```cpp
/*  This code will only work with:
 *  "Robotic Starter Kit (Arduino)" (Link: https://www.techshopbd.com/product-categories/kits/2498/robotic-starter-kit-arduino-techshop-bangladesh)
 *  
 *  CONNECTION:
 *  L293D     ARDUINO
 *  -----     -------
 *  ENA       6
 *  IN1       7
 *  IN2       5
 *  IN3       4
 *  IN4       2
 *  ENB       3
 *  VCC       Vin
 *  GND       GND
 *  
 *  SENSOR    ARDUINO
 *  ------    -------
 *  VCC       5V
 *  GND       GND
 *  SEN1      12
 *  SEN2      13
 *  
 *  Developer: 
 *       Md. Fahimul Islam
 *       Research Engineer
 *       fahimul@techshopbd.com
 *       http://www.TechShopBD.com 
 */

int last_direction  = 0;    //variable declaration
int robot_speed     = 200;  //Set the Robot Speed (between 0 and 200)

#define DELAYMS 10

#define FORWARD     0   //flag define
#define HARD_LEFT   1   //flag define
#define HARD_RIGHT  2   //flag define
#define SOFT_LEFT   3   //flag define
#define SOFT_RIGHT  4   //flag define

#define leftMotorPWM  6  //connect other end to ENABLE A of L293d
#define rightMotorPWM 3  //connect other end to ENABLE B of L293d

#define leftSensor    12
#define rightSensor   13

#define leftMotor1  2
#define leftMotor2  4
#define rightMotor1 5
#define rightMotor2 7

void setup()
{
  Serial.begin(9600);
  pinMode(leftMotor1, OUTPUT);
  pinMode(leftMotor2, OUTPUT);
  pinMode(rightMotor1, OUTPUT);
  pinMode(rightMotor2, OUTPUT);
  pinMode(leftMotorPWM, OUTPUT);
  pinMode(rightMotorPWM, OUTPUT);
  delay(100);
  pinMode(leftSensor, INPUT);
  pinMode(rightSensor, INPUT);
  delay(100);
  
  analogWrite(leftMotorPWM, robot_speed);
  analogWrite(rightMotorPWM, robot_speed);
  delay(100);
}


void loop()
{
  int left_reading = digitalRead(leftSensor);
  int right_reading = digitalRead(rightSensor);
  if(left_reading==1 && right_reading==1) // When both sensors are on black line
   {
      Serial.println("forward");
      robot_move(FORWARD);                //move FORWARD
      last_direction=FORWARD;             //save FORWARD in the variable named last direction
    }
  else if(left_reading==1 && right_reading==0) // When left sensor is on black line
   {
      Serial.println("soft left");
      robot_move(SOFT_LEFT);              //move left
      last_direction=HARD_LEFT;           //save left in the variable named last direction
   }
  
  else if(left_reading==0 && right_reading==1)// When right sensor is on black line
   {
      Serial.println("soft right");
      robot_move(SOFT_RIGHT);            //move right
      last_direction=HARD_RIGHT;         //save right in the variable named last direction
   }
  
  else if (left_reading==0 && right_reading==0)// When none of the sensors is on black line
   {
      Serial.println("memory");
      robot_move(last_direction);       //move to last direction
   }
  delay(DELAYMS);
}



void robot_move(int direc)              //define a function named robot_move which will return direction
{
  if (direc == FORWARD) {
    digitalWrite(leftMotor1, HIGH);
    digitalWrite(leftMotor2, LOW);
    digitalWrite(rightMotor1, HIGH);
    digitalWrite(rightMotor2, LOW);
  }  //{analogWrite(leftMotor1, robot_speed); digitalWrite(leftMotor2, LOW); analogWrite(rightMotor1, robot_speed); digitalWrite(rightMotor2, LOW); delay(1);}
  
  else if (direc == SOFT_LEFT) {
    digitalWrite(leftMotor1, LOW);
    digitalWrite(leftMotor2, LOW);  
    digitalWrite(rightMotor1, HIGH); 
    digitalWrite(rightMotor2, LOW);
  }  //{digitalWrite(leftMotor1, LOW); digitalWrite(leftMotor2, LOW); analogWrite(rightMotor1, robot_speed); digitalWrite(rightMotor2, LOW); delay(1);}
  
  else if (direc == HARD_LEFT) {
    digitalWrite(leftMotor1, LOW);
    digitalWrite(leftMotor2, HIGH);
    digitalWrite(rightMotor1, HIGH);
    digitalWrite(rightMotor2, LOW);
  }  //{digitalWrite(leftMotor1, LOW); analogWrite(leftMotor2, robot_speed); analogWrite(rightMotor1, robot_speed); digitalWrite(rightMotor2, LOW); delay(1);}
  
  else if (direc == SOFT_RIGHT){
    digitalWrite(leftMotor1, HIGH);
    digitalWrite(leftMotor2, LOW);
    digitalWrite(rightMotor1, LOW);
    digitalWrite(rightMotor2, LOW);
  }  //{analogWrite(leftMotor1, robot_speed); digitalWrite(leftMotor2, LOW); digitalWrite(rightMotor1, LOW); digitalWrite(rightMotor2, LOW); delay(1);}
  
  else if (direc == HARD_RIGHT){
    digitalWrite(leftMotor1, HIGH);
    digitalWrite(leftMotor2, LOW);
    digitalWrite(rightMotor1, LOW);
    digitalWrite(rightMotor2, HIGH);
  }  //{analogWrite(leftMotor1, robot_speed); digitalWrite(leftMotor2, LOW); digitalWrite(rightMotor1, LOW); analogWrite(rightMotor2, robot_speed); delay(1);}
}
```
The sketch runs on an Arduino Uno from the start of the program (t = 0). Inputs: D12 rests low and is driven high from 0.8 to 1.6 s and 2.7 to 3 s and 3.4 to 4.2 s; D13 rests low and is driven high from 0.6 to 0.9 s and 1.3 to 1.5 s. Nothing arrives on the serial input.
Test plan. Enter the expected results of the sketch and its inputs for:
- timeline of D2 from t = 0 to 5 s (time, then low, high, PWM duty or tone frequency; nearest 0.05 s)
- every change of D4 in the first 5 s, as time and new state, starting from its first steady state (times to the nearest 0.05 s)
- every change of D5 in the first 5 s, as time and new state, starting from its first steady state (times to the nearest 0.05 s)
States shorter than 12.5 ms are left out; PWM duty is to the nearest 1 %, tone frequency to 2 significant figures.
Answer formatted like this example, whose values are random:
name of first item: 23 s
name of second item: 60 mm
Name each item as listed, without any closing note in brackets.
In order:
timeline of D2 from t = 0 to 5 s: 0 s low; 0.3 s high; 0.9 s low; 1.3 s high; 1.5 s low
every change of D4 in the first 5 s, as time and new state, starting from its first steady state: 0 s low; 1.6 s high; 2.7 s low; 3 s high; 3.4 s low; 4.2 s high
every change of D5 in the first 5 s, as time and new state, starting from its first steady state: 0 s low; 0.3 s high; 0.6 s low; 0.8 s high
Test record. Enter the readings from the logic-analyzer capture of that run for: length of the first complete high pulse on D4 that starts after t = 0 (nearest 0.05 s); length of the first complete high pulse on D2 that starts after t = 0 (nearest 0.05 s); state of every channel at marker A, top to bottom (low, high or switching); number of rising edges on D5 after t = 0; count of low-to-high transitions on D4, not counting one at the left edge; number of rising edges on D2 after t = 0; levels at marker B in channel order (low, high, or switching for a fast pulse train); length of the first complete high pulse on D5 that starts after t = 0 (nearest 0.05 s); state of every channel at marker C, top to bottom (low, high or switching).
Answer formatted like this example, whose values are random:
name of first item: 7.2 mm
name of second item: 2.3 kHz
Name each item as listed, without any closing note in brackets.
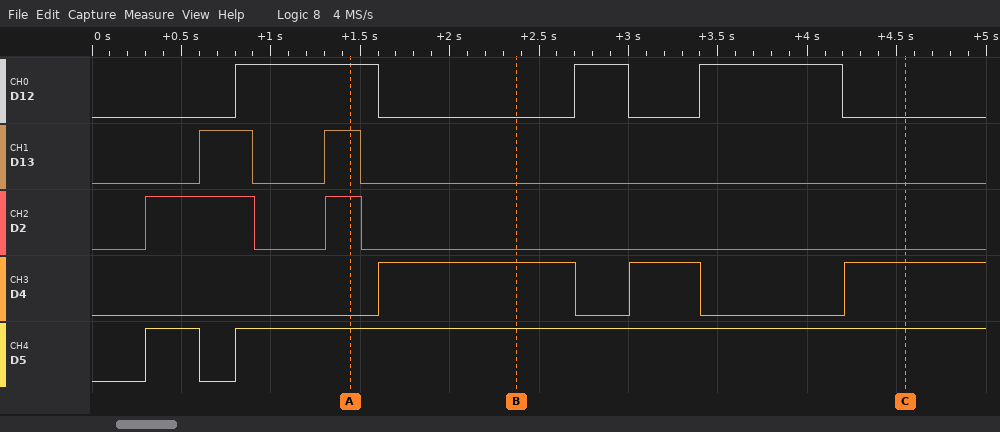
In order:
length of the first complete high pulse on D4 that starts after t = 0: 1.10 s
length of the first complete high pulse on D2 that starts after t = 0: 0.60 s
state of every channel at marker A, top to bottom: D12 high, D13 high, D2 high, D4 low, D5 high
number of rising edges on D5 after t = 0: 2
count of low-to-high transitions on D4, not counting one at the left edge: 3
number of rising edges on D2 after t = 0: 2
levels at marker B in channel order: D12 low, D13 low, D2 low, D4 high, D5 high
length of the first complete high pulse on D5 that starts after t = 0: 0.30 s
state of every channel at marker C, top to bottom: D12 low, D13 low, D2 low, D4 high, D5 high
